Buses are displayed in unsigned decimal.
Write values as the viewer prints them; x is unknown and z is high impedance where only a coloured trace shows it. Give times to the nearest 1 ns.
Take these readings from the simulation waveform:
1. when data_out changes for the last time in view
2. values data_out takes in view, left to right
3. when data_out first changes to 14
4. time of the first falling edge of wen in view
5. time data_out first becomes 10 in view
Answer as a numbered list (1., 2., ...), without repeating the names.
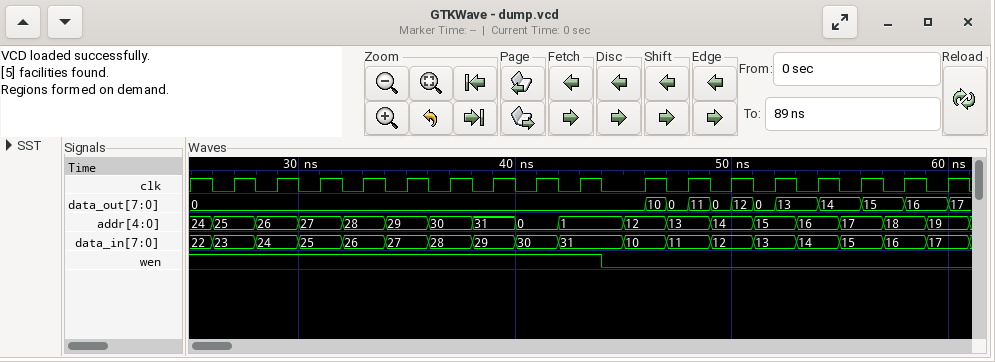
1. 60 ns
2. 0, 10, 0, 11, 0, 12, 0, 13, 14, 15, 16, 17
3. 54 ns
4. 44 ns
5. 46 ns
